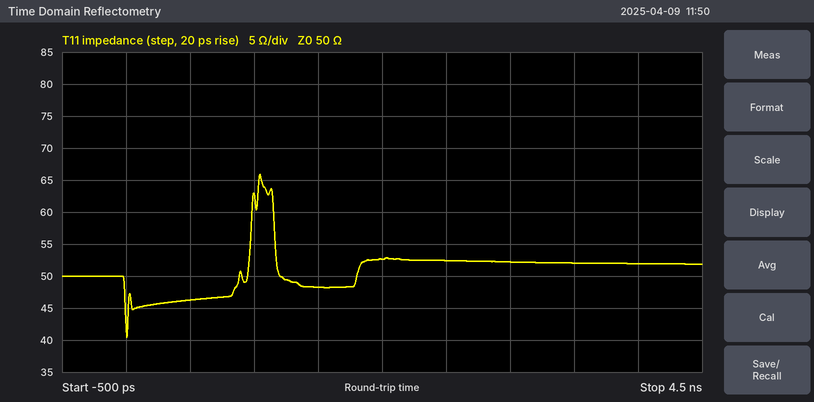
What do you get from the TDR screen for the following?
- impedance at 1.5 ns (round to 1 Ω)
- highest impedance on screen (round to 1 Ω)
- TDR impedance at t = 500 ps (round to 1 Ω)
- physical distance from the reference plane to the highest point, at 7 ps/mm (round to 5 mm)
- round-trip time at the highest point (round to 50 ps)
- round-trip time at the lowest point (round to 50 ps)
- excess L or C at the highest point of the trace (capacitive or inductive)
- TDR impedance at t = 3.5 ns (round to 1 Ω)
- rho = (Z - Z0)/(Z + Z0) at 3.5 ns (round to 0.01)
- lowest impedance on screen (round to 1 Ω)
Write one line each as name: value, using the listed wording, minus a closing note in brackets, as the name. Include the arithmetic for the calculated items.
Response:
impedance at 1.5 ns: 48 Ω
highest impedance on screen: 66 Ω
TDR impedance at t = 500 ps: 46 Ω
physical distance from the reference plane to the highest point, at 7 ps/mm: 1.05 ns / 2 / 7 ps/mm ≈ 75 mm
round-trip time at the highest point: 1.05 ns
round-trip time at the lowest point: 0 ps
excess L or C at the highest point of the trace: inductive
TDR impedance at t = 3.5 ns: 52 Ω
rho = (Z - Z0)/(Z + Z0) at 3.5 ns: (52 − 50)/(52 + 50) ≈ +0.02
lowest impedance on screen: 40 Ω
